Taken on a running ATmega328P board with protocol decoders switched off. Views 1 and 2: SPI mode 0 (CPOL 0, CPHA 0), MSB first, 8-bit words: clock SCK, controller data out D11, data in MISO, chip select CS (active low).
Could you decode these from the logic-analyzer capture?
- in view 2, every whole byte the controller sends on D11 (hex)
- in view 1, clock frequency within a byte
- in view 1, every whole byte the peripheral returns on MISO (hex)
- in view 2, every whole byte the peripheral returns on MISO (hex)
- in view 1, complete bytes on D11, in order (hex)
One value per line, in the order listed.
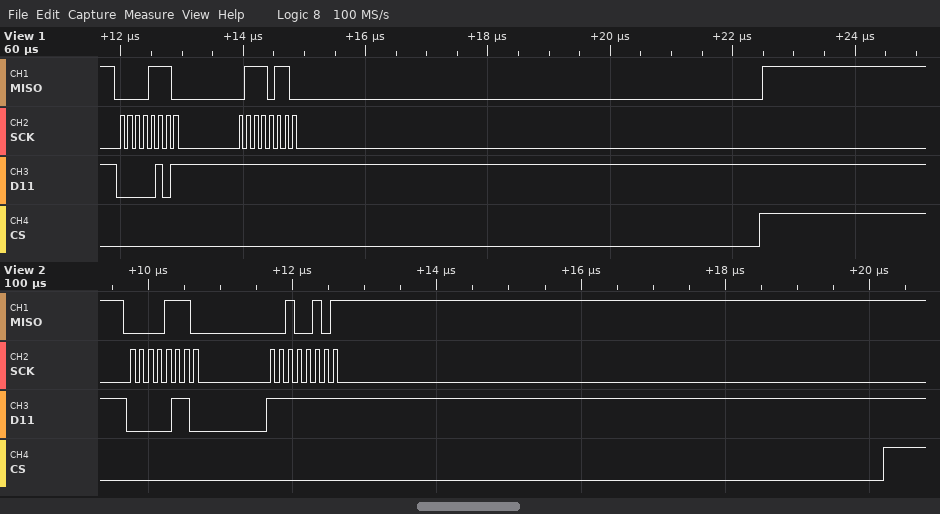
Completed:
0x06 0xFF
8 MHz
0E 76
0x0E 0x25
05 FF
